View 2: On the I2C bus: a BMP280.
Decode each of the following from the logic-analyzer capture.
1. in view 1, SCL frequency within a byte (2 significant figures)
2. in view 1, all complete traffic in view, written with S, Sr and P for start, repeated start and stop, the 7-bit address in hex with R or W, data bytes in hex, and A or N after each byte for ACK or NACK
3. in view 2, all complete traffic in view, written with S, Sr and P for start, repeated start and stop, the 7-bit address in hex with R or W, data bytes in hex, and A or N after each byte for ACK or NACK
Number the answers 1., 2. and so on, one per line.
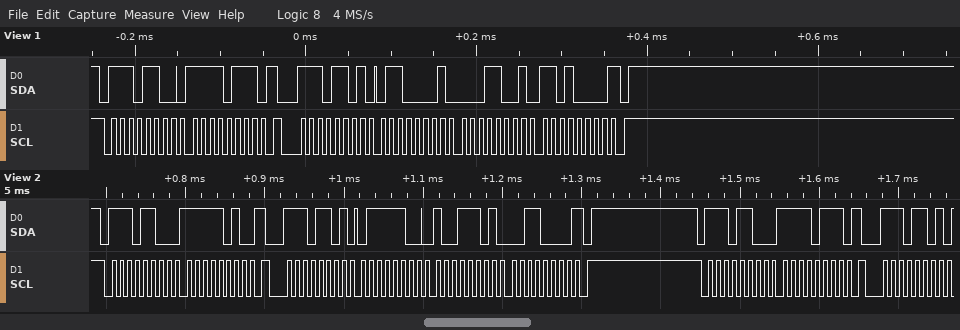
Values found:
1. 100 kHz
2. S 76W A F7 A Sr 76R A 61 A 19 A D0 N P
3. S 76W A FA A Sr 76R A 7C A 9D A 30 N P S 76W A F7 A Sr 76R A
